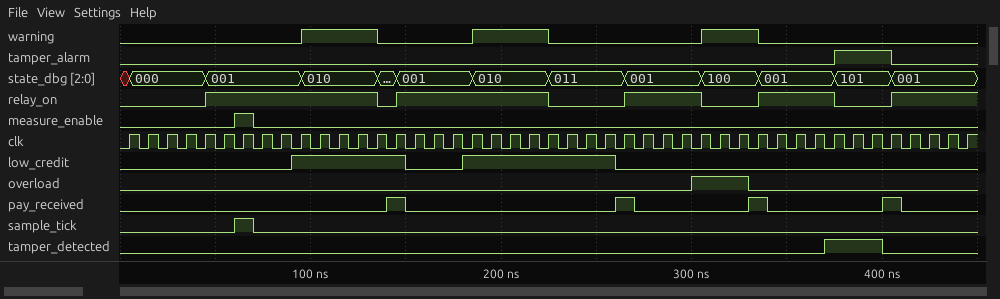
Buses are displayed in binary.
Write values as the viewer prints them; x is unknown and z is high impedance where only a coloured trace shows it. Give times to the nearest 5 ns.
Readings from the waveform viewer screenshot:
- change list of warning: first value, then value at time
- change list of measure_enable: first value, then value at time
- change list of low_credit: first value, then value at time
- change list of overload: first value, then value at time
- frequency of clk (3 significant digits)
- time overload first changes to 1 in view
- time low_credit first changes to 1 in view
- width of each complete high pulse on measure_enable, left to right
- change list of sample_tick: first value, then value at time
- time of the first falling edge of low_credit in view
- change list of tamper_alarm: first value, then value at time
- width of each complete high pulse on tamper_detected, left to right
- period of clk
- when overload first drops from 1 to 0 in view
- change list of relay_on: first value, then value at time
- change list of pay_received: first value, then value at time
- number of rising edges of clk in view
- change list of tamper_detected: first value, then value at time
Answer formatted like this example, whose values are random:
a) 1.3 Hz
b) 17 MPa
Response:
a) 0, 1 at 95 ns, 0 at 135 ns, 1 at 185 ns, 0 at 225 ns, 1 at 305 ns, 0 at 335 ns
b) 0, 1 at 60 ns, 0 at 70 ns
c) 0, 1 at 90 ns, 0 at 150 ns, 1 at 180 ns, 0 at 260 ns
d) 0, 1 at 300 ns, 0 at 330 ns
e) 100 MHz
f) 300 ns
g) 90 ns
h) 10 ns
i) 0, 1 at 60 ns, 0 at 70 ns
j) 150 ns
k) 0, 1 at 375 ns, 0 at 405 ns
l) 30 ns
m) 10 ns
n) 330 ns
o) 0, 1 at 45 ns, 0 at 135 ns, 1 at 145 ns, 0 at 225 ns, 1 at 265 ns, 0 at 305 ns, 1 at 335 ns, 0 at 375 ns, 1 at 405 ns
p) 0, 1 at 140 ns, 0 at 150 ns, 1 at 260 ns, 0 at 270 ns, 1 at 330 ns, 0 at 340 ns, 1 at 400 ns, 0 at 410 ns
q) 45
r) 0, 1 at 370 ns, 0 at 400 ns
